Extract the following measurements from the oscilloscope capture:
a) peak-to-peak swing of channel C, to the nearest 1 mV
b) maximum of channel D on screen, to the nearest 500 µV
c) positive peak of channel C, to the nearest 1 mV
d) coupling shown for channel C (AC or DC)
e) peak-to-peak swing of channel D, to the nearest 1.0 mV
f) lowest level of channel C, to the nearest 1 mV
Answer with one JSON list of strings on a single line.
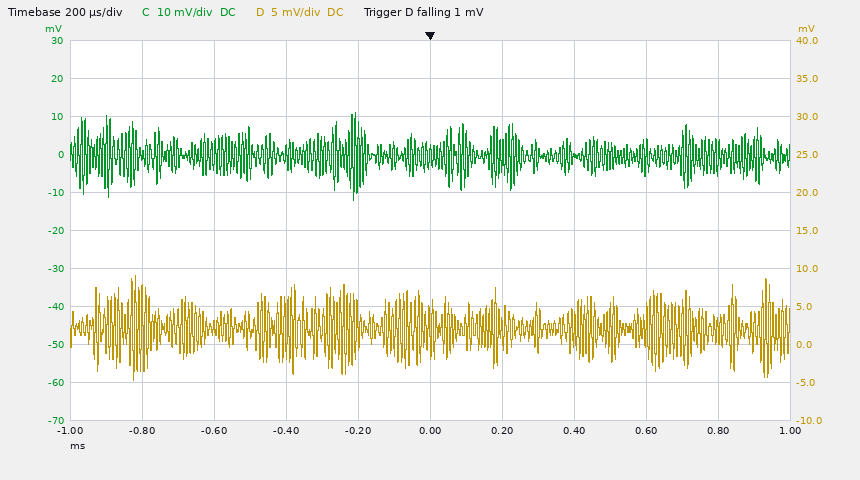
["23 mV", "9.0 mV", "11 mV", "DC", "14.0 mV", "-12 mV"]
